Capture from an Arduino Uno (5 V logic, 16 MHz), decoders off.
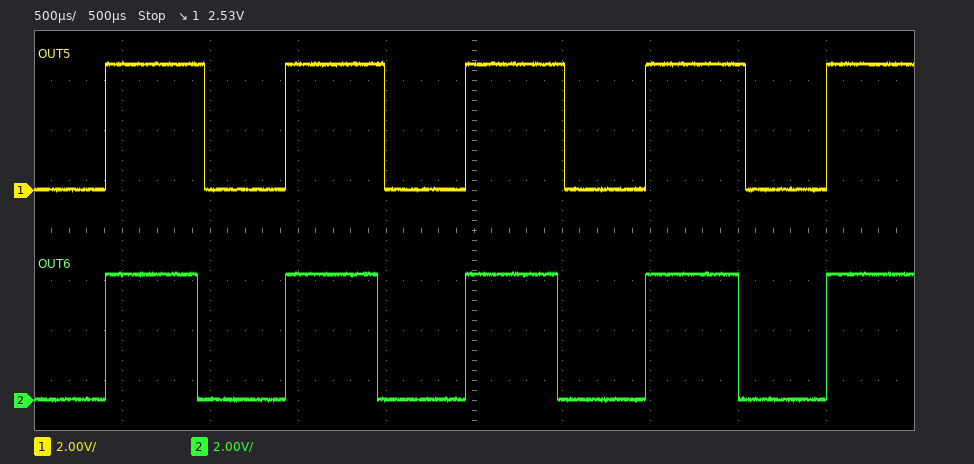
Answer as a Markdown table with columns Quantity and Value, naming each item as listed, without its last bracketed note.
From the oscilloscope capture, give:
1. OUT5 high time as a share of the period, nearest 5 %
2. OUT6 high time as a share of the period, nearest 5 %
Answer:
| Quantity | Value |
|---|---|
| OUT5 high time as a share of the period, nearest 5 % | 55 % |
| OUT6 high time as a share of the period, nearest 5 % | 50 % |
